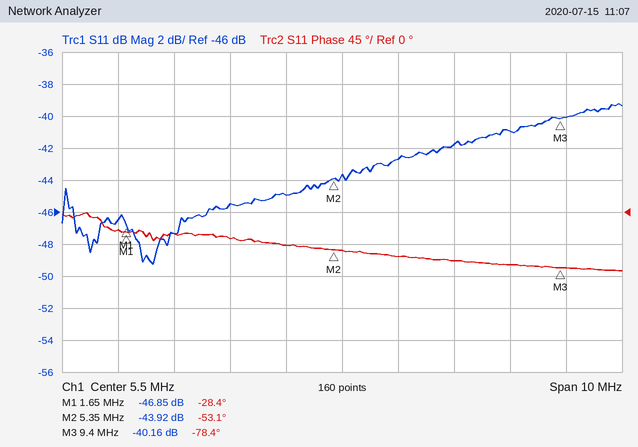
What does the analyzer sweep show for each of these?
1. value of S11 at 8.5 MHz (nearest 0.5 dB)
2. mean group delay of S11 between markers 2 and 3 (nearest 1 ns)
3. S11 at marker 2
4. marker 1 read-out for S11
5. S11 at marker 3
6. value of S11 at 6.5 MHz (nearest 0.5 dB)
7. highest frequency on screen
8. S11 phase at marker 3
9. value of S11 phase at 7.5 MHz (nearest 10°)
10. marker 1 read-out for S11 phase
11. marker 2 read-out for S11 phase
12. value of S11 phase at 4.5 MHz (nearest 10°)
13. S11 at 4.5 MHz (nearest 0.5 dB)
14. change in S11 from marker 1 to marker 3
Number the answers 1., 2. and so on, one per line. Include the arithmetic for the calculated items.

1. -41.0 dB
2. −(-78.4° − (-53.1°))/(360° × 4.05 MHz) ≈ 17 ns
3. -43.92 dB
4. -46.85 dB
5. -40.16 dB
6. -42.5 dB
7. 10.5 MHz
8. -78.4°
9. -70°
10. -28.4°
11. -53.1°
12. -50°
13. -45.0 dB
14. -40.16 − (-46.85) = 6.69 dB
